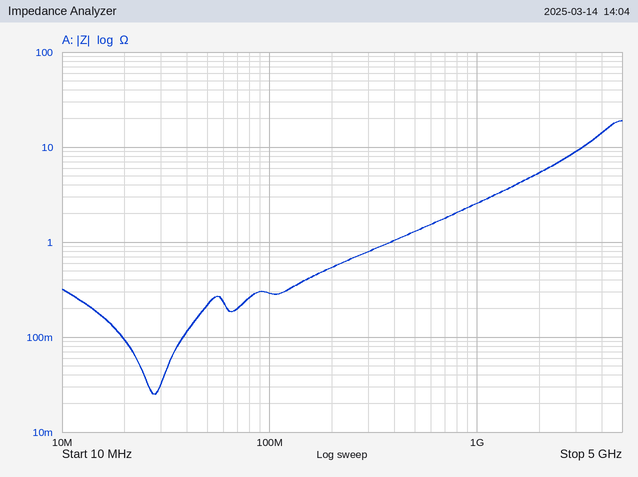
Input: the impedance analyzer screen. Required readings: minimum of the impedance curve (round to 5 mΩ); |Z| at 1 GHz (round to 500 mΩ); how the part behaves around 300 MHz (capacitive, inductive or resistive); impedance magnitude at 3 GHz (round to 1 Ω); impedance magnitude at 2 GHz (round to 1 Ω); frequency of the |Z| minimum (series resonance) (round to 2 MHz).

25 mΩ
2.5 Ω
inductive
9 Ω
5 Ω
28 MHz
